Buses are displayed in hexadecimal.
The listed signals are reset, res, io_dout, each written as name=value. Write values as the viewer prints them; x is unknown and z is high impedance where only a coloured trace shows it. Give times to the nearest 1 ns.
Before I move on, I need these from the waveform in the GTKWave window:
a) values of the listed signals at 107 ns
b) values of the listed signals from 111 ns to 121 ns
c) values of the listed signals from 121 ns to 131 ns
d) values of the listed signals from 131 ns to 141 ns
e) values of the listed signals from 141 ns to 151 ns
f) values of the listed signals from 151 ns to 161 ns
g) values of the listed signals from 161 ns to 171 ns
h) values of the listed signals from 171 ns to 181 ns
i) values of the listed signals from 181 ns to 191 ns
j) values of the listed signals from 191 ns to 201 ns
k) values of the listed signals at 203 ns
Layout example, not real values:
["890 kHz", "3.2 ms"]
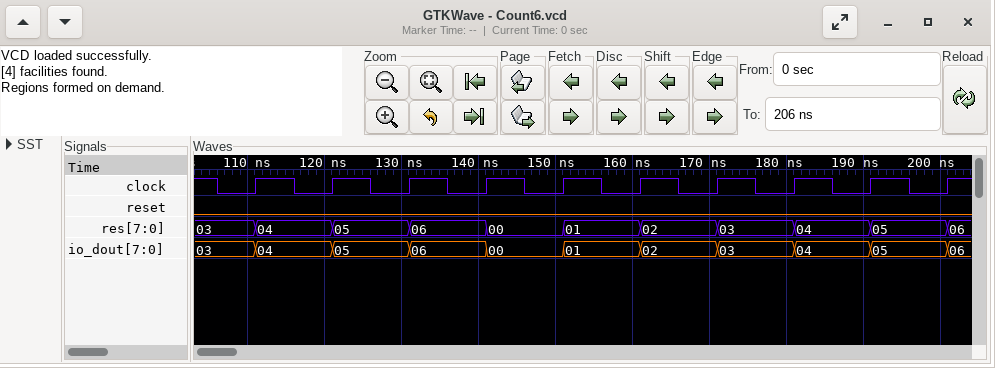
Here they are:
["reset=0, res=03, io_dout=03", "reset=0, res=04, io_dout=04", "reset=0, res=05, io_dout=05", "reset=0, res=06, io_dout=06", "reset=0, res=00, io_dout=00", "reset=0, res=01, io_dout=01", "reset=0, res=02, io_dout=02", "reset=0, res=03, io_dout=03", "reset=0, res=04, io_dout=04", "reset=0, res=05, io_dout=05", "reset=0, res=06, io_dout=06"]
